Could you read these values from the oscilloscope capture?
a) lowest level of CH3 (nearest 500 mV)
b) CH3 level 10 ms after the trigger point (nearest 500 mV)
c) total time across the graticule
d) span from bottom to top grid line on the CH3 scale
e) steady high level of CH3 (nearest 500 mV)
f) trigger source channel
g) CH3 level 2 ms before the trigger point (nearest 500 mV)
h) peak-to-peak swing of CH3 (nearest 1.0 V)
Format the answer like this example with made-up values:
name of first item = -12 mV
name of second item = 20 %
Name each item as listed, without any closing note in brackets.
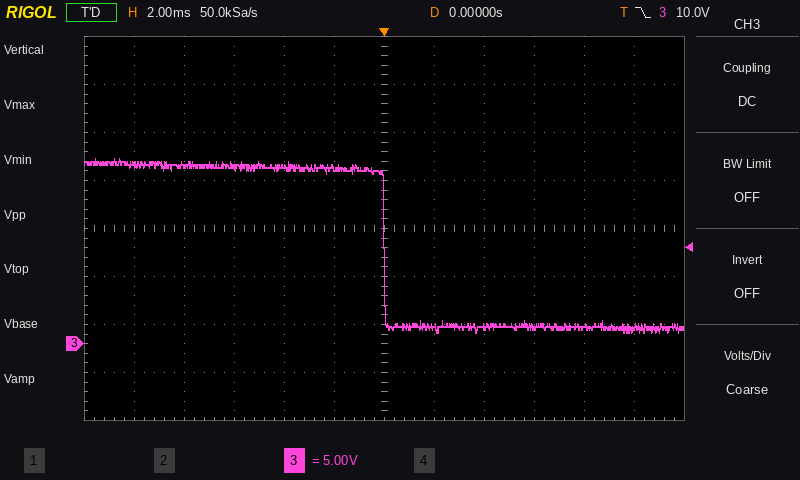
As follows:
lowest level of CH3 = 1.0 V
CH3 level 10 ms after the trigger point = 1.5 V
total time across the graticule = 24 ms
span from bottom to top grid line on the CH3 scale = 40 V
steady high level of CH3 = 18.5 V
trigger source channel = CH3
CH3 level 2 ms before the trigger point = 18.5 V
peak-to-peak swing of CH3 = 18.0 V
